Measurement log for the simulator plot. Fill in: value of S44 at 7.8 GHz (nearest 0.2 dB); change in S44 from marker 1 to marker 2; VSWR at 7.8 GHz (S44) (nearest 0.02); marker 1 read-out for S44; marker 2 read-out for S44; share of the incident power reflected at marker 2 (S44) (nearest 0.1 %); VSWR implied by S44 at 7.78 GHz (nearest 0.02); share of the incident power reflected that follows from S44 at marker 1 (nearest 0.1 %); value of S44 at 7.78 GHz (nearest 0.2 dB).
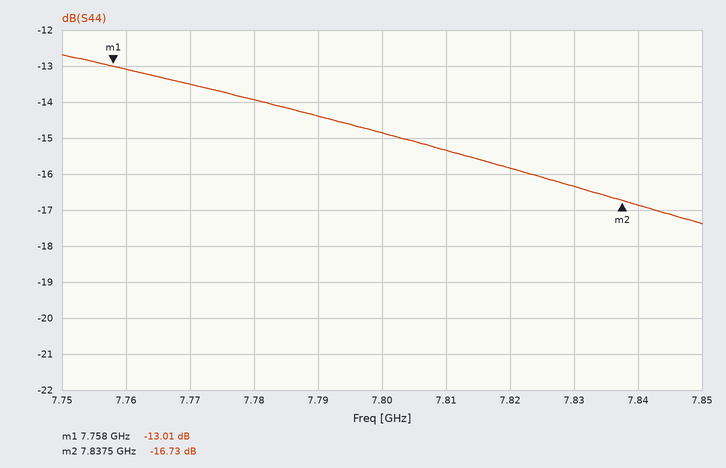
-14.8 dB
-3.72 dB
1.44
-13.01 dB
-16.73 dB
2.1 %
1.50
5.0 %
-14.0 dB
